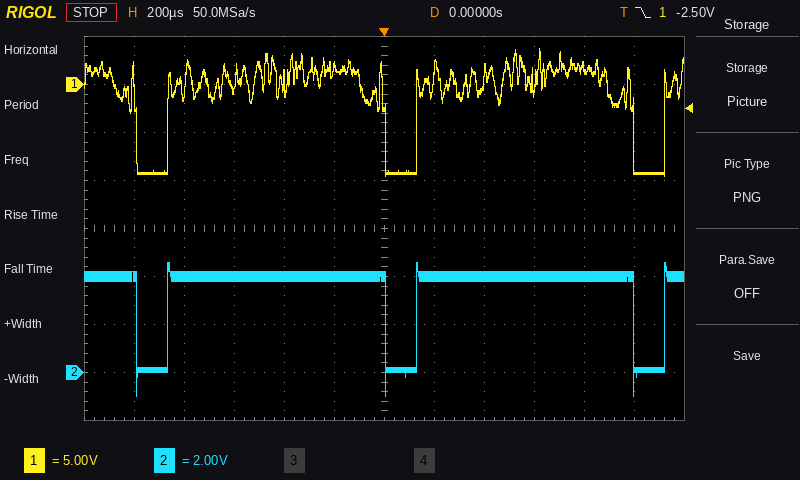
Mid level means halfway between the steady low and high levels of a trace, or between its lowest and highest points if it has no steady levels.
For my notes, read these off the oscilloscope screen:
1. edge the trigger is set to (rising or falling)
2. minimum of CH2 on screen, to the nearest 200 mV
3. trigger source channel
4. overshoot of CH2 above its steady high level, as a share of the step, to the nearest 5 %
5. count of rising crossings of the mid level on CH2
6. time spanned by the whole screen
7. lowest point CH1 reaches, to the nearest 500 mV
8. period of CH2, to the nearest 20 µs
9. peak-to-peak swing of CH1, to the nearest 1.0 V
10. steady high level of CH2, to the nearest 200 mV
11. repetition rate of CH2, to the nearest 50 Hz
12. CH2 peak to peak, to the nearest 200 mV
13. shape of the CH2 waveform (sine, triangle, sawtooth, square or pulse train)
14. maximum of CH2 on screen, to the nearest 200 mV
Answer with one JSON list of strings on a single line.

["falling", "-1.0 V", "CH1", "15 %", "3", "2.4 ms", "-9.5 V", "1.00 ms", "13.0 V", "4.0 V", "1.00 kHz", "5.6 V", "pulse train", "4.6 V"]
